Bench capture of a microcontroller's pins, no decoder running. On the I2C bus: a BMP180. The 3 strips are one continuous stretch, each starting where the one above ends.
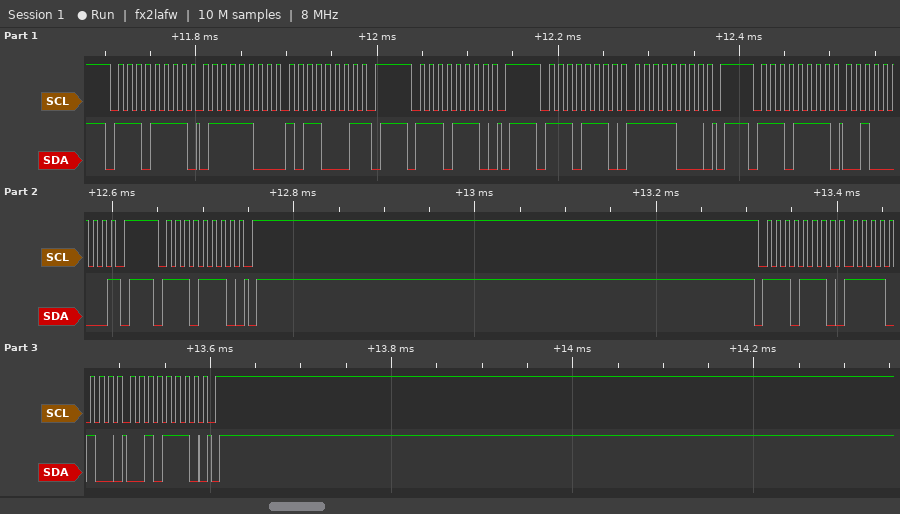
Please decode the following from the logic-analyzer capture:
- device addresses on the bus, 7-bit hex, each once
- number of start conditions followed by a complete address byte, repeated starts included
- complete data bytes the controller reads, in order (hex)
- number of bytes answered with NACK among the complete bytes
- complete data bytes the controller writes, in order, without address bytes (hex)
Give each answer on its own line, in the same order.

0x77
6
7C B1 20
2
F8 F4 2E
